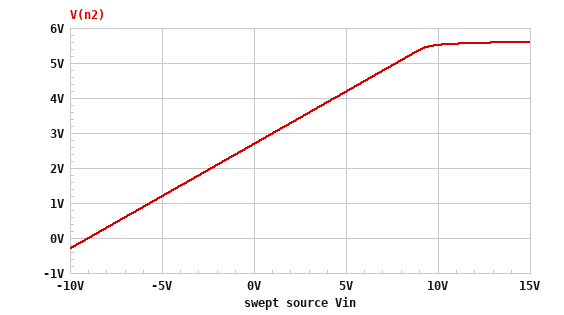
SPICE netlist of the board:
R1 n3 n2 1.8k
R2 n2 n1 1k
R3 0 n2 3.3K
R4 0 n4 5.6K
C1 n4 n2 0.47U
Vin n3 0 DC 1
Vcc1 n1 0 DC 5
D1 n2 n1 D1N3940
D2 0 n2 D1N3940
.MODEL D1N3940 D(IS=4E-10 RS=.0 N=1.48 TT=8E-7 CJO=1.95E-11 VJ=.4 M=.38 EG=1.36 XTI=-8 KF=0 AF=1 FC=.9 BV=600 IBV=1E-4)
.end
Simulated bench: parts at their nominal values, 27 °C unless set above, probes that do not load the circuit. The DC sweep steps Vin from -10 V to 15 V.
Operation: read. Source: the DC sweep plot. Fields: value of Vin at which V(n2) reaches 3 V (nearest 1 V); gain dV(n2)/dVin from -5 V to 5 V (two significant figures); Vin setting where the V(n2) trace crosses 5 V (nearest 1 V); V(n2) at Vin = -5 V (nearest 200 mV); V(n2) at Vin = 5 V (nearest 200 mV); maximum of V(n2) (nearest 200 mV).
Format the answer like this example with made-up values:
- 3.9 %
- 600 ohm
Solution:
- 1 V
- 0.30 V/V
- 8 V
- 1.2 V
- 4.2 V
- 5.6 V
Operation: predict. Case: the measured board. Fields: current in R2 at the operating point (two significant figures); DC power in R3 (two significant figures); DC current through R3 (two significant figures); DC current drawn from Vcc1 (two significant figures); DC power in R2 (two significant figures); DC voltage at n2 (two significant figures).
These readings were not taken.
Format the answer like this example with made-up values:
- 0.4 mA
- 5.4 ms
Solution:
- 2.0 mA
- 2.7 mW
- 910 µA
- 2.0 mA
- 4.0 mW
- 3.0 V
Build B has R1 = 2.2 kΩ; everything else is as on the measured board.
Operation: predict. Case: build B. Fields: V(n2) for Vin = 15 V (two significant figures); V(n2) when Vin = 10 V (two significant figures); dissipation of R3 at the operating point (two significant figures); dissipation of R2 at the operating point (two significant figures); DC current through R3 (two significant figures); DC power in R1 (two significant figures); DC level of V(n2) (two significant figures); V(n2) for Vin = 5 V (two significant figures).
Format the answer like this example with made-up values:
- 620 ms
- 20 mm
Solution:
- 5.6 V
- 5.4 V
- 2.9 mW
- 3.6 mW
- 940 µA
- 2.0 mW
- 3.1 V
- 4.1 V
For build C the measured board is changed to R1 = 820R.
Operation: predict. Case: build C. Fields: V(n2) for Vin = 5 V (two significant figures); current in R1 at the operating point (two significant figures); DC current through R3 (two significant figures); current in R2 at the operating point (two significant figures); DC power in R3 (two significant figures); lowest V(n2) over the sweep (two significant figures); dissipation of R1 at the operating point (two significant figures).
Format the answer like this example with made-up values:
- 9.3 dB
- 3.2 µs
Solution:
- 4.4 V
- 1.8 mA
- 750 µA
- 2.5 mA
- 1.8 mW
- -630 mV
- 2.6 mW
